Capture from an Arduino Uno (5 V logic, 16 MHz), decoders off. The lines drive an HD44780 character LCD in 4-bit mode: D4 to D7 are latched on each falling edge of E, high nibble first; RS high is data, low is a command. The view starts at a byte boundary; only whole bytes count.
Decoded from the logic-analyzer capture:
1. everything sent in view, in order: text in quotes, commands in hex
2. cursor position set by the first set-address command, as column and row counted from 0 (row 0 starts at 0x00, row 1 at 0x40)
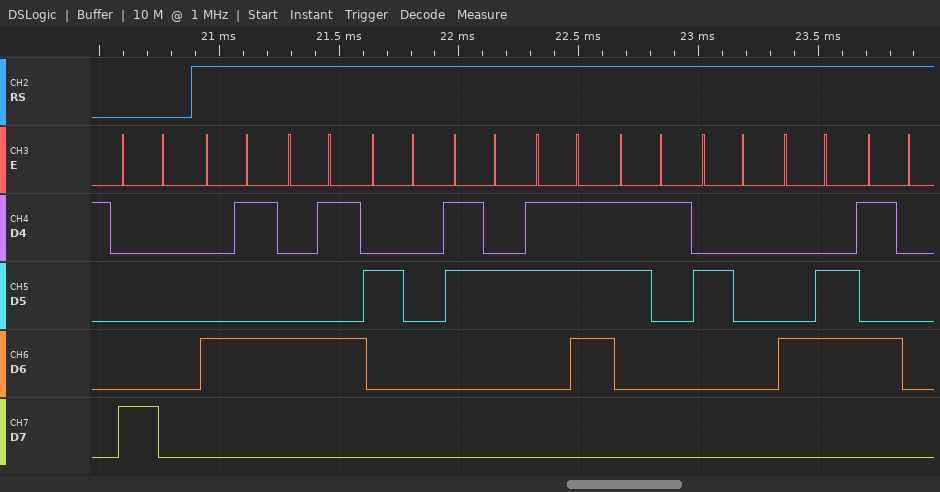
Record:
0x80 "EE 271 FP"
column 0, row 0
